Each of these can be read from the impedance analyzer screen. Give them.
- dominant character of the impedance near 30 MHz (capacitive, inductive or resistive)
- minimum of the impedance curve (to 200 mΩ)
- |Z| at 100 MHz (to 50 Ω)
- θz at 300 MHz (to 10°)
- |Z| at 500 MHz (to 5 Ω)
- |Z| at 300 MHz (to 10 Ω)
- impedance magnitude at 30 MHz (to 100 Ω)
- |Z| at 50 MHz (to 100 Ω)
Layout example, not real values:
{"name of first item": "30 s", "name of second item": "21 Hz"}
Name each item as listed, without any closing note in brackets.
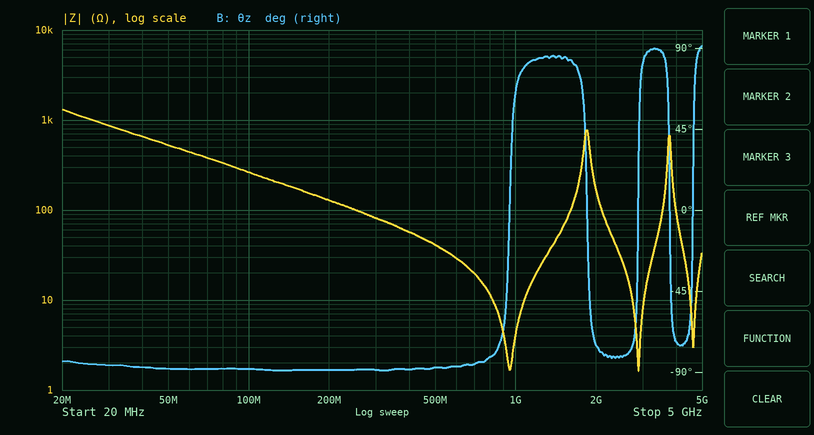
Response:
{"dominant character of the impedance near 30 MHz": "capacitive", "minimum of the impedance curve": "1.6 Ω", "|Z| at 100 MHz": "250 Ω", "θz at 300 MHz": "-90°", "|Z| at 500 MHz": "40 Ω", "|Z| at 300 MHz": "80 Ω", "impedance magnitude at 30 MHz": "900 Ω", "|Z| at 50 MHz": "500 Ω"}
